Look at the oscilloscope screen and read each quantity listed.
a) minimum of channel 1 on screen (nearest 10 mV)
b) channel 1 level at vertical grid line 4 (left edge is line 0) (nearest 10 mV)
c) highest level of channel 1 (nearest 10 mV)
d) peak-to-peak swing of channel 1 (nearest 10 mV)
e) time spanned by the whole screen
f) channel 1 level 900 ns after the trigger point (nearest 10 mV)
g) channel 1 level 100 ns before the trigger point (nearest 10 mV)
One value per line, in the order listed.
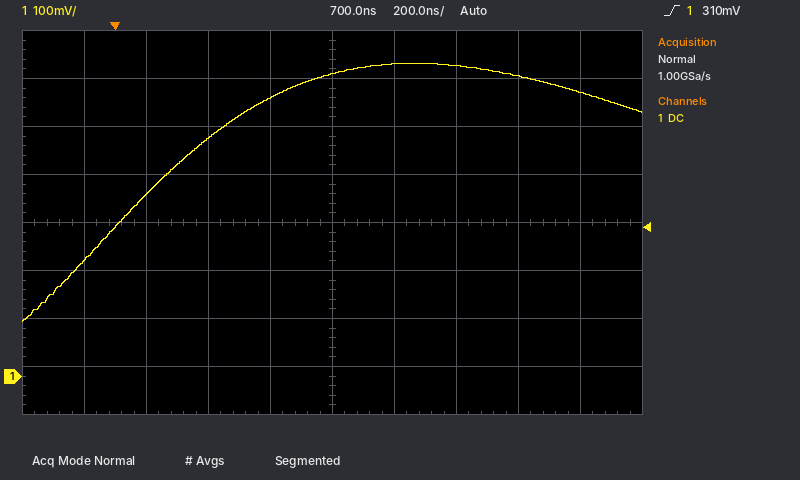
110 mV
580 mV
650 mV
540 mV
2 µs
650 mV
240 mV
